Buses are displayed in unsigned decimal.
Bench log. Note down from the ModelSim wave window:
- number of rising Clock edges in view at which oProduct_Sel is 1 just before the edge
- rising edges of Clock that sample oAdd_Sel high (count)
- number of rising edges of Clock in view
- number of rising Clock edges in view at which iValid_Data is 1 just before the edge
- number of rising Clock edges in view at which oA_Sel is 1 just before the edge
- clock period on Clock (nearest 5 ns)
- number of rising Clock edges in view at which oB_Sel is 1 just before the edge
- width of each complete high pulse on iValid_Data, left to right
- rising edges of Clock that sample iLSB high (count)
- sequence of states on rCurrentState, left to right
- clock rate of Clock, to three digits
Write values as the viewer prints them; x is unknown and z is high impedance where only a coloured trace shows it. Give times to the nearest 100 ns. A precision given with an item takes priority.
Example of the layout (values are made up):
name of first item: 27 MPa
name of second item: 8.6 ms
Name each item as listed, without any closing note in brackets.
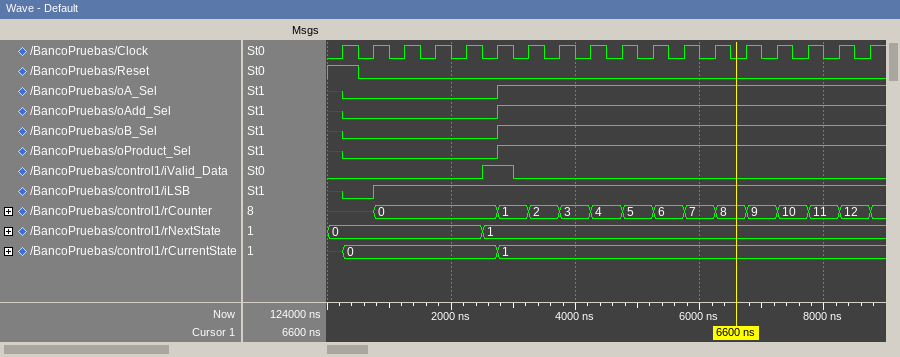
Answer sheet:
number of rising Clock edges in view at which oProduct_Sel is 1 just before the edge: 12
rising edges of Clock that sample oAdd_Sel high: 12
number of rising edges of Clock in view: 18
number of rising Clock edges in view at which iValid_Data is 1 just before the edge: 1
number of rising Clock edges in view at which oA_Sel is 1 just before the edge: 12
clock period on Clock: 500 ns
number of rising Clock edges in view at which oB_Sel is 1 just before the edge: 12
width of each complete high pulse on iValid_Data, left to right: 500 ns
rising edges of Clock that sample iLSB high: 16
sequence of states on rCurrentState, left to right: x, 0, 1
clock rate of Clock, to three digits: 2.00 MHz
